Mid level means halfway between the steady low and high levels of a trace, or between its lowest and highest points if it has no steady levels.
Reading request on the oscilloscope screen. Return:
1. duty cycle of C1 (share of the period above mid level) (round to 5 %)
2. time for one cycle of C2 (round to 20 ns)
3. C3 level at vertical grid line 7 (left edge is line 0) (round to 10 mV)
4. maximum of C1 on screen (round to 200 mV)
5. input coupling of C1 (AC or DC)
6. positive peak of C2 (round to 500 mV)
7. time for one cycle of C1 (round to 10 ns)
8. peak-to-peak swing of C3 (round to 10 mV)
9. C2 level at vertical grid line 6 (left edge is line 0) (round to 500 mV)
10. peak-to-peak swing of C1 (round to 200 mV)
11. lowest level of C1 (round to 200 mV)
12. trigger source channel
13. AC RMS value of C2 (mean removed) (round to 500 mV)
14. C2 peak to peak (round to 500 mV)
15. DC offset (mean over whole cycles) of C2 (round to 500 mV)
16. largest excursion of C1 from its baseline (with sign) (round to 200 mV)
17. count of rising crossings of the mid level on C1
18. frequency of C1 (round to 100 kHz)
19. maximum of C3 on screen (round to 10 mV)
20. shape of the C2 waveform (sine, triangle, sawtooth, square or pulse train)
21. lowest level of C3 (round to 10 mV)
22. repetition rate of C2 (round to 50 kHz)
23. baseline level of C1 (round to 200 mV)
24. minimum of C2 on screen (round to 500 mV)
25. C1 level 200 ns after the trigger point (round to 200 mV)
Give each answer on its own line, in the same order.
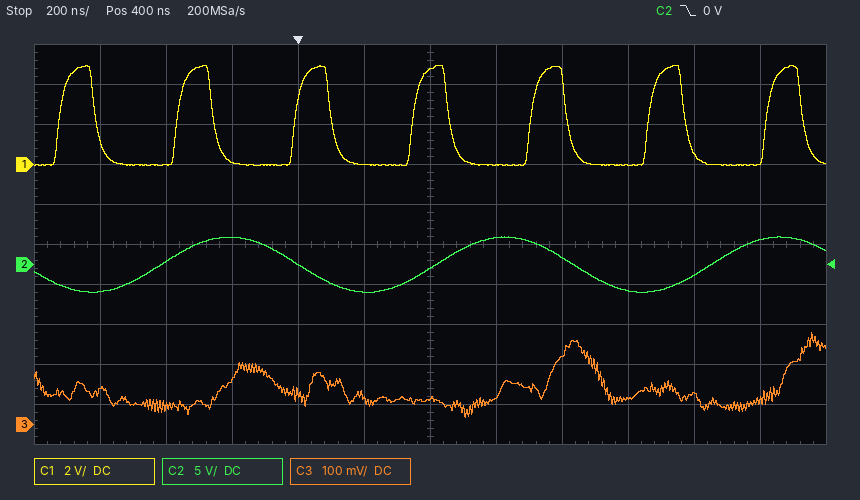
30 %
840 ns
70 mV
5.0 V
DC
3.5 V
360 ns
210 mV
-500 mV
5.0 V
0.0 V
C2
2.5 V
7.0 V
0.0 V
+5.0 V
7
2.8 MHz
230 mV
sine
20 mV
1.20 MHz
0.0 V
-3.5 V
0.0 V
